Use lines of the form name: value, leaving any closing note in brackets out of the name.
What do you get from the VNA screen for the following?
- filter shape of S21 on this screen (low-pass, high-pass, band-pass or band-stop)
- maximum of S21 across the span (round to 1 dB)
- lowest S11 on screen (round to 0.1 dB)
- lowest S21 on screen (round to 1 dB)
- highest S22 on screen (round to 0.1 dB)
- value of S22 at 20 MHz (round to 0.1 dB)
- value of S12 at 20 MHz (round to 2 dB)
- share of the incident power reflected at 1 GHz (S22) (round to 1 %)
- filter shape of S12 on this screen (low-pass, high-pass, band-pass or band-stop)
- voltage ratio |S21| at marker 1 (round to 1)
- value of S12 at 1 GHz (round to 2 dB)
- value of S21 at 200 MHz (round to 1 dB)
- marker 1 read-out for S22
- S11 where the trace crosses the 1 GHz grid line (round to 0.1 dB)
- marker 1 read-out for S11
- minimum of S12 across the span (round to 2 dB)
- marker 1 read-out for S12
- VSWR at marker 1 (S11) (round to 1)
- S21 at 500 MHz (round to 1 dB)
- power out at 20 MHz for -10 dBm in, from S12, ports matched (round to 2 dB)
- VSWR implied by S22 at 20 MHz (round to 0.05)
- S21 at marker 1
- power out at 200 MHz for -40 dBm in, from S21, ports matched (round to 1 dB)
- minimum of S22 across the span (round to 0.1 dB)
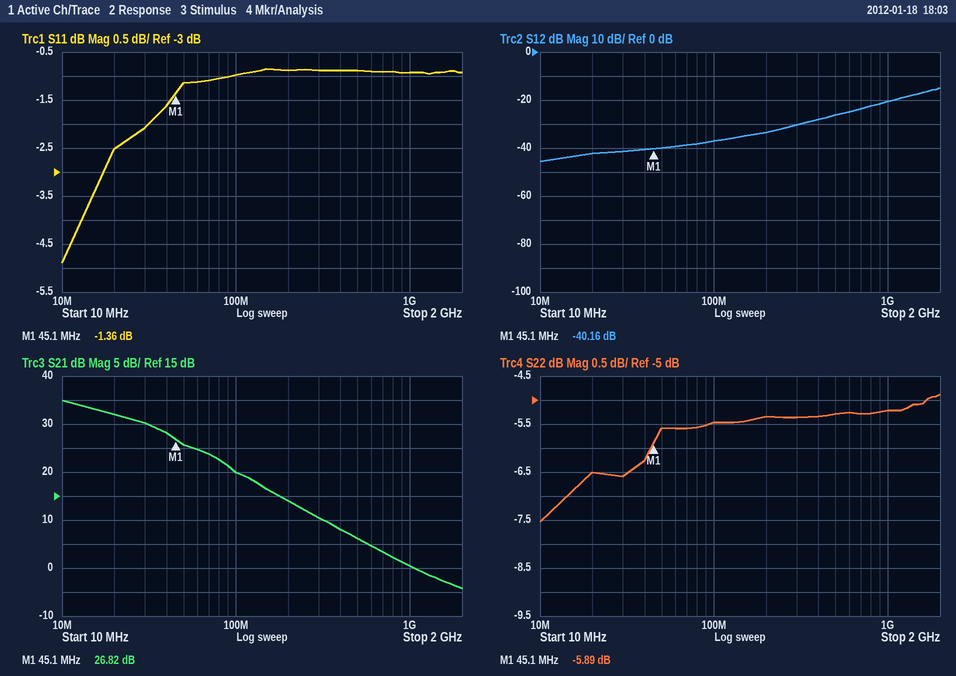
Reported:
filter shape of S21 on this screen: low-pass
maximum of S21 across the span: 35 dB
lowest S11 on screen: -4.9 dB
lowest S21 on screen: -4 dB
highest S22 on screen: -4.9 dB
value of S22 at 20 MHz: -6.5 dB
value of S12 at 20 MHz: -42 dB
share of the incident power reflected at 1 GHz (S22): 30 %
filter shape of S12 on this screen: high-pass
voltage ratio |S21| at marker 1: 22
value of S12 at 1 GHz: -20 dB
value of S21 at 200 MHz: 14 dB
marker 1 read-out for S22: -5.89 dB
S11 where the trace crosses the 1 GHz grid line: -0.9 dB
marker 1 read-out for S11: -1.36 dB
minimum of S12 across the span: -46 dB
marker 1 read-out for S12: -40.16 dB
VSWR at marker 1 (S11): 13
S21 at 500 MHz: 6 dB
power out at 20 MHz for -10 dBm in, from S12, ports matched: -52 dBm
VSWR implied by S22 at 20 MHz: 2.80
S21 at marker 1: 26.82 dB
power out at 200 MHz for -40 dBm in, from S21, ports matched: -26 dBm
minimum of S22 across the span: -7.5 dB
